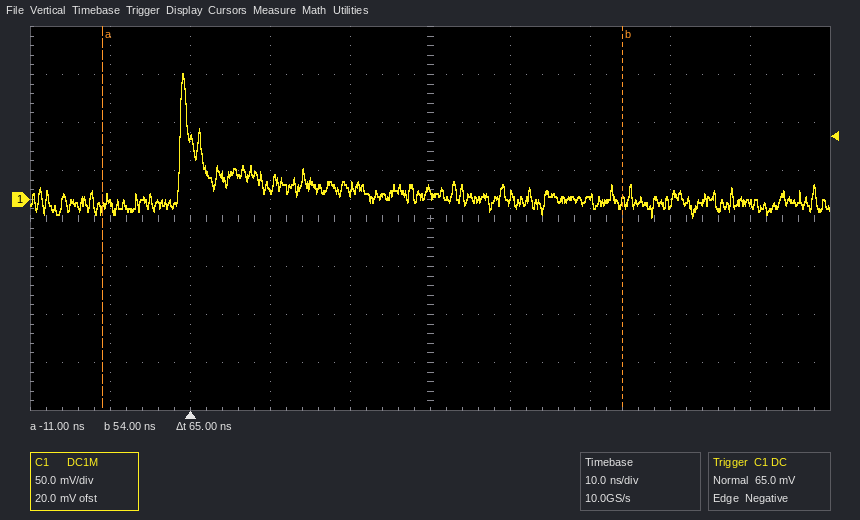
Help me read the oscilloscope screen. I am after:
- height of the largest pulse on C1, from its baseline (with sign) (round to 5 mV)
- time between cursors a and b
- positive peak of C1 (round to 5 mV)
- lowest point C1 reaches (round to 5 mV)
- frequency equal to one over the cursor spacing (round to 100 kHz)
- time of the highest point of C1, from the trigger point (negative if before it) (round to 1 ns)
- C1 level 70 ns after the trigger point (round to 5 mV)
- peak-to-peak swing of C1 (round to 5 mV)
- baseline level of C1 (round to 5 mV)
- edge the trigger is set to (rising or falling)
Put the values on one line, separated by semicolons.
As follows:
+130 mV; 65 ns; 130 mV; -20 mV; 15.4 MHz; -1 ns; -5 mV; 150 mV; 0 mV; falling
